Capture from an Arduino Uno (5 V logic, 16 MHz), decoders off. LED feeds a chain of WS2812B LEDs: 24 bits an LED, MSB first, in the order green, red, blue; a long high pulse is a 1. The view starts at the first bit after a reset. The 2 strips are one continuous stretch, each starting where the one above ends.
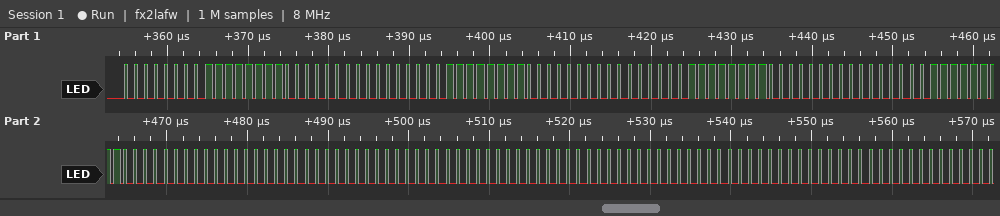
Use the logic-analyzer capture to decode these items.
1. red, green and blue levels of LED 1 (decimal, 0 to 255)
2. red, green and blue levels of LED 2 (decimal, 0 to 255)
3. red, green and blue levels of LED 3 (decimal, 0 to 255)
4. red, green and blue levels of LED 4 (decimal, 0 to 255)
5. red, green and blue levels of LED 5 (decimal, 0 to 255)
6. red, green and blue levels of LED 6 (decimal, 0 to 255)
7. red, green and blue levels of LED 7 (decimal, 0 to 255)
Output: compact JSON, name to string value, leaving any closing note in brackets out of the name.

{"red, green and blue levels of LED 1": "255, 0, 0", "red, green and blue levels of LED 2": "255, 0, 0", "red, green and blue levels of LED 3": "255, 0, 0", "red, green and blue levels of LED 4": "255, 0, 0", "red, green and blue levels of LED 5": "0, 0, 0", "red, green and blue levels of LED 6": "0, 0, 0", "red, green and blue levels of LED 7": "0, 0, 0"}
